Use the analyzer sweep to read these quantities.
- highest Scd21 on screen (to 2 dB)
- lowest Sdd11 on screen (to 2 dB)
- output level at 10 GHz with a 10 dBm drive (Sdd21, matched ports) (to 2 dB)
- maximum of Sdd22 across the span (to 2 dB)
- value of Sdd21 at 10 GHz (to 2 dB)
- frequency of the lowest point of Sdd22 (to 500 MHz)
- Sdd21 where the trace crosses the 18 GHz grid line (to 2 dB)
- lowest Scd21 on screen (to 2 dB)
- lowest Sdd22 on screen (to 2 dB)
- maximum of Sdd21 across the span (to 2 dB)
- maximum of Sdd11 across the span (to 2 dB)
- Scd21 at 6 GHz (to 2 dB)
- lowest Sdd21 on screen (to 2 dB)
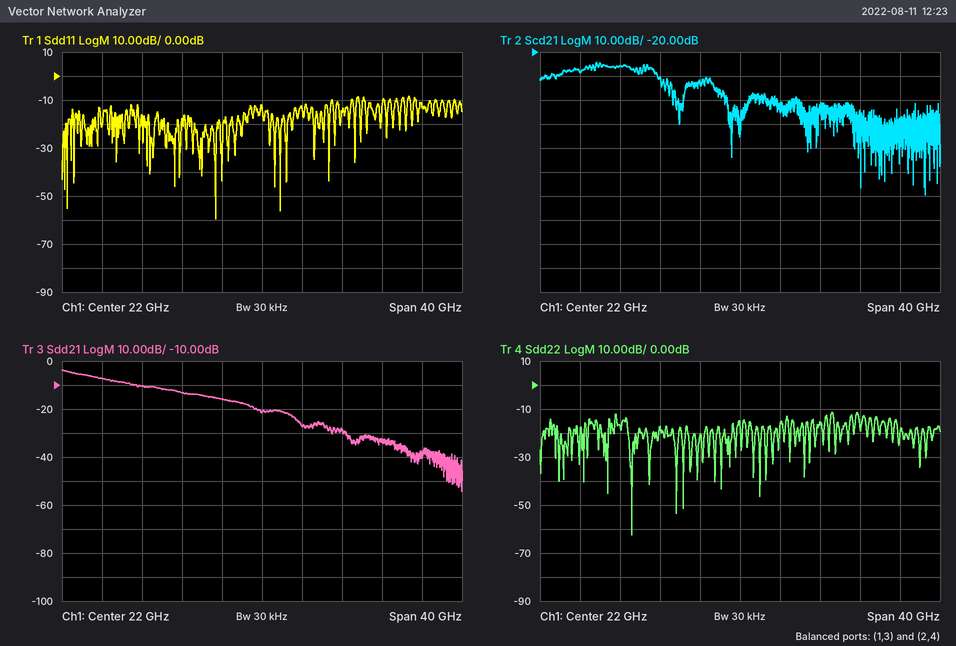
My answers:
-24 dB
-60 dB
0 dBm
-12 dB
-10 dB
11.0 GHz
-16 dB
-80 dB
-62 dB
-4 dB
-8 dB
-28 dB
-54 dB
